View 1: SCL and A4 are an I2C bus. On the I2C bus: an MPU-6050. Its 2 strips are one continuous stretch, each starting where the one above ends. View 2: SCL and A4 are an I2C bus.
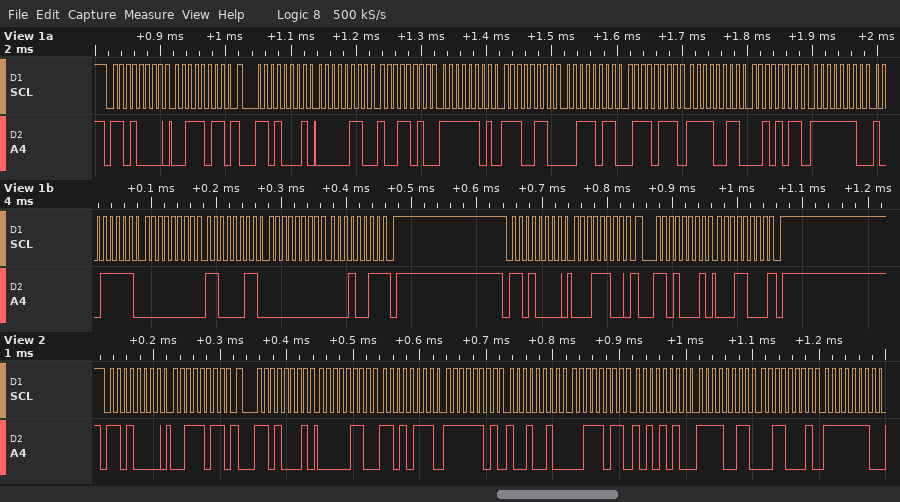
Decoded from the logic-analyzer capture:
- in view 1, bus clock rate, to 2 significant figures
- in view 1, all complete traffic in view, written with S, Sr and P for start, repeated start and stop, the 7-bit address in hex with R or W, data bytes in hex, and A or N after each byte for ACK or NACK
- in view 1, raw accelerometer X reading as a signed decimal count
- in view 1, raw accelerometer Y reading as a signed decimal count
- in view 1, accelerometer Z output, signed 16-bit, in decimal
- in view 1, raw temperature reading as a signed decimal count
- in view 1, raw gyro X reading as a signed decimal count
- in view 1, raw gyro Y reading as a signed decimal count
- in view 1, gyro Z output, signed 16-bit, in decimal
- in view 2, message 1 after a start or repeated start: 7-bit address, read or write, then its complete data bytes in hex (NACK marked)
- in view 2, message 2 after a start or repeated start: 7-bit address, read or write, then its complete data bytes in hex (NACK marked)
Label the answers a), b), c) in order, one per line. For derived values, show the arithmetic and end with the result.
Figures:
a) 100 kHz
b) S 68W A 3B A Sr 68R A 06 A 9A A FD A E6 A 3B A 77 A F3 A 2B A FE A 9F A 00 A C3 A 00 A 13 N P S 68W A 1C A Sr 68R A 18 N P
c) 0x069A = 1690
d) 0xFDE6 = -538
e) 0x3B77 = 15223
f) 0xF32B = -3285
g) 0xFE9F = -353
h) 0x00C3 = 195
i) 0x0013 = 19
j) 0x68 write: 3B
k) 0x68 read: 06 D7 FD 92 3B AA F3 31 FE
